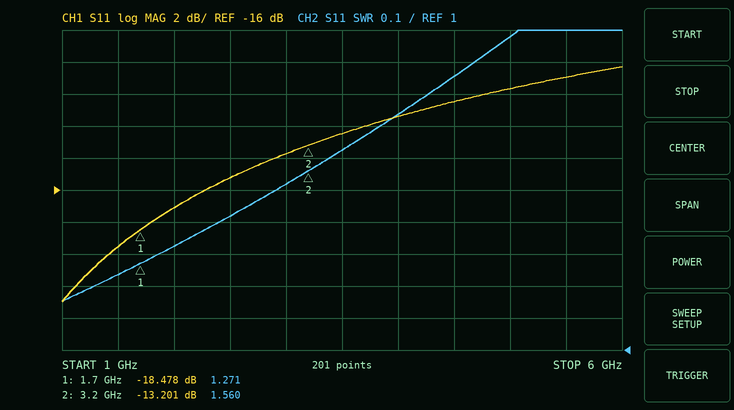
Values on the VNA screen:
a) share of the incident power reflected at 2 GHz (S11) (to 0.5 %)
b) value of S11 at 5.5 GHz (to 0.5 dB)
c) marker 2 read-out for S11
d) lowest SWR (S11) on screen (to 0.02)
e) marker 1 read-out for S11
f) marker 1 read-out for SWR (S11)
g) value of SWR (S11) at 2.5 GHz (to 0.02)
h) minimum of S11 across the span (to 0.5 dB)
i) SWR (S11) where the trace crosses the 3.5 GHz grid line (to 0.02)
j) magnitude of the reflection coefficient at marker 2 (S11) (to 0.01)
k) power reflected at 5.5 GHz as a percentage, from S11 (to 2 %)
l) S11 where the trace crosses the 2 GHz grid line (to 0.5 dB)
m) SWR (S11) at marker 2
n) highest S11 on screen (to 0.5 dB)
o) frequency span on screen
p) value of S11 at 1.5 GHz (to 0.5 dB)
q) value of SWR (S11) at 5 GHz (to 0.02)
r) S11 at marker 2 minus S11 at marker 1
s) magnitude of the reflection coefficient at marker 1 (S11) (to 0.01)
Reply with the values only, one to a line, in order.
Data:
2.0 %
-9.0 dB
-13.201 dB
1.16
-18.478 dB
1.271
1.42
-23.0 dB
1.62
0.22
12 %
-17.0 dB
1.560
-8.5 dB
5 GHz
-19.5 dB
1.98
5.277 dB
0.12
